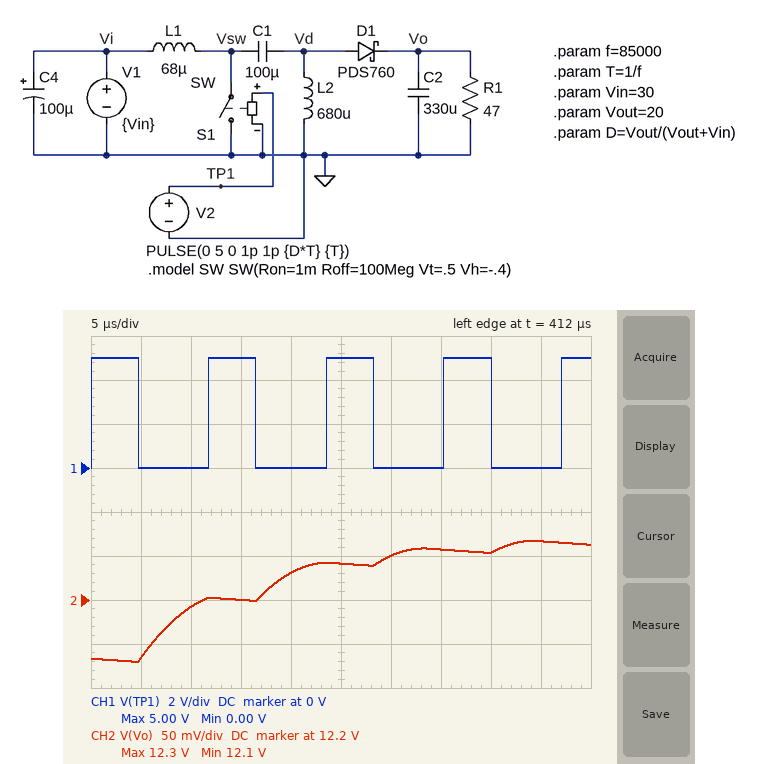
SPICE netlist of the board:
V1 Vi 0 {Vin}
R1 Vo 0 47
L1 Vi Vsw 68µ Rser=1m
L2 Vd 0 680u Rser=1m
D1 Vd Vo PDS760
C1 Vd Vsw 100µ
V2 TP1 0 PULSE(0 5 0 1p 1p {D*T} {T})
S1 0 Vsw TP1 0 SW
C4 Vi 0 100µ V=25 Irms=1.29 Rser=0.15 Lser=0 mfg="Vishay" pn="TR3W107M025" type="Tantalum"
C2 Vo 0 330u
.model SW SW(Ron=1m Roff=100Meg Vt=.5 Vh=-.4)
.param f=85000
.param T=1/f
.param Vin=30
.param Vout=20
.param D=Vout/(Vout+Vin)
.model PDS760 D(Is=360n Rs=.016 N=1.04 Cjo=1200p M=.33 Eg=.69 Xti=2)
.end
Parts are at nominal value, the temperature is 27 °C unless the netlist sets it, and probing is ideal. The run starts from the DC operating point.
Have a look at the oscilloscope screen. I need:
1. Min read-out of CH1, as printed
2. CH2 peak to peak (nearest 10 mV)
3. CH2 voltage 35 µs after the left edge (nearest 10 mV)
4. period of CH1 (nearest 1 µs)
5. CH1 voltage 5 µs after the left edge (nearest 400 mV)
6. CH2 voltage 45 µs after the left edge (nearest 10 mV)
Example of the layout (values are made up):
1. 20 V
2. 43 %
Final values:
1. 0.00 V
2. 140 mV
3. 12.26 V
4. 12 µs
5. 0 V
6. 12.27 V
